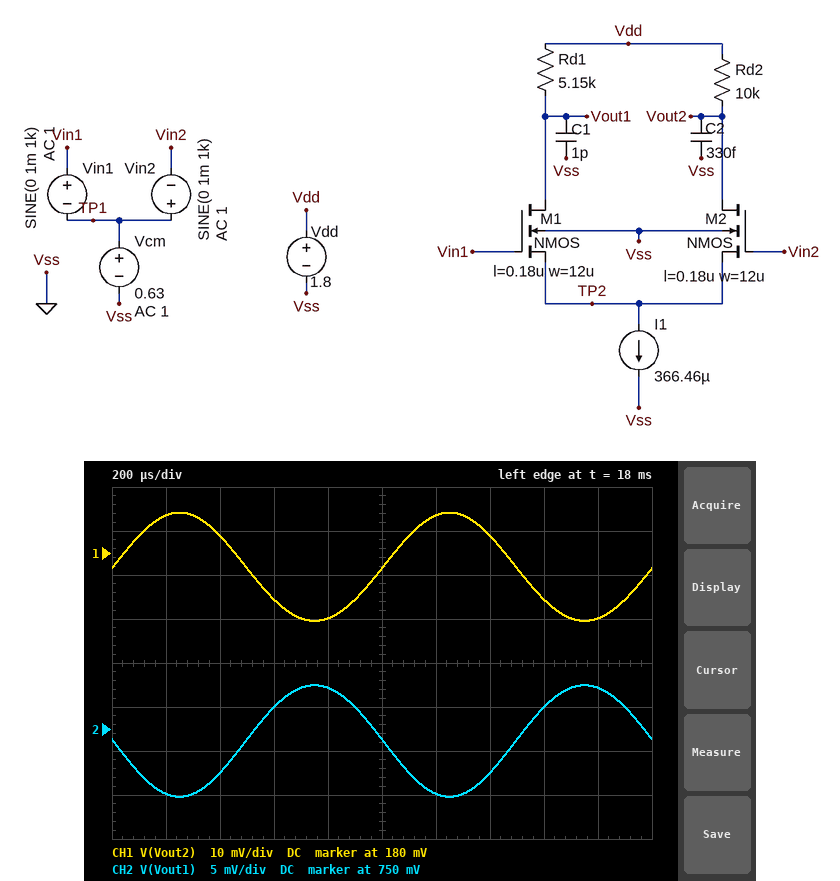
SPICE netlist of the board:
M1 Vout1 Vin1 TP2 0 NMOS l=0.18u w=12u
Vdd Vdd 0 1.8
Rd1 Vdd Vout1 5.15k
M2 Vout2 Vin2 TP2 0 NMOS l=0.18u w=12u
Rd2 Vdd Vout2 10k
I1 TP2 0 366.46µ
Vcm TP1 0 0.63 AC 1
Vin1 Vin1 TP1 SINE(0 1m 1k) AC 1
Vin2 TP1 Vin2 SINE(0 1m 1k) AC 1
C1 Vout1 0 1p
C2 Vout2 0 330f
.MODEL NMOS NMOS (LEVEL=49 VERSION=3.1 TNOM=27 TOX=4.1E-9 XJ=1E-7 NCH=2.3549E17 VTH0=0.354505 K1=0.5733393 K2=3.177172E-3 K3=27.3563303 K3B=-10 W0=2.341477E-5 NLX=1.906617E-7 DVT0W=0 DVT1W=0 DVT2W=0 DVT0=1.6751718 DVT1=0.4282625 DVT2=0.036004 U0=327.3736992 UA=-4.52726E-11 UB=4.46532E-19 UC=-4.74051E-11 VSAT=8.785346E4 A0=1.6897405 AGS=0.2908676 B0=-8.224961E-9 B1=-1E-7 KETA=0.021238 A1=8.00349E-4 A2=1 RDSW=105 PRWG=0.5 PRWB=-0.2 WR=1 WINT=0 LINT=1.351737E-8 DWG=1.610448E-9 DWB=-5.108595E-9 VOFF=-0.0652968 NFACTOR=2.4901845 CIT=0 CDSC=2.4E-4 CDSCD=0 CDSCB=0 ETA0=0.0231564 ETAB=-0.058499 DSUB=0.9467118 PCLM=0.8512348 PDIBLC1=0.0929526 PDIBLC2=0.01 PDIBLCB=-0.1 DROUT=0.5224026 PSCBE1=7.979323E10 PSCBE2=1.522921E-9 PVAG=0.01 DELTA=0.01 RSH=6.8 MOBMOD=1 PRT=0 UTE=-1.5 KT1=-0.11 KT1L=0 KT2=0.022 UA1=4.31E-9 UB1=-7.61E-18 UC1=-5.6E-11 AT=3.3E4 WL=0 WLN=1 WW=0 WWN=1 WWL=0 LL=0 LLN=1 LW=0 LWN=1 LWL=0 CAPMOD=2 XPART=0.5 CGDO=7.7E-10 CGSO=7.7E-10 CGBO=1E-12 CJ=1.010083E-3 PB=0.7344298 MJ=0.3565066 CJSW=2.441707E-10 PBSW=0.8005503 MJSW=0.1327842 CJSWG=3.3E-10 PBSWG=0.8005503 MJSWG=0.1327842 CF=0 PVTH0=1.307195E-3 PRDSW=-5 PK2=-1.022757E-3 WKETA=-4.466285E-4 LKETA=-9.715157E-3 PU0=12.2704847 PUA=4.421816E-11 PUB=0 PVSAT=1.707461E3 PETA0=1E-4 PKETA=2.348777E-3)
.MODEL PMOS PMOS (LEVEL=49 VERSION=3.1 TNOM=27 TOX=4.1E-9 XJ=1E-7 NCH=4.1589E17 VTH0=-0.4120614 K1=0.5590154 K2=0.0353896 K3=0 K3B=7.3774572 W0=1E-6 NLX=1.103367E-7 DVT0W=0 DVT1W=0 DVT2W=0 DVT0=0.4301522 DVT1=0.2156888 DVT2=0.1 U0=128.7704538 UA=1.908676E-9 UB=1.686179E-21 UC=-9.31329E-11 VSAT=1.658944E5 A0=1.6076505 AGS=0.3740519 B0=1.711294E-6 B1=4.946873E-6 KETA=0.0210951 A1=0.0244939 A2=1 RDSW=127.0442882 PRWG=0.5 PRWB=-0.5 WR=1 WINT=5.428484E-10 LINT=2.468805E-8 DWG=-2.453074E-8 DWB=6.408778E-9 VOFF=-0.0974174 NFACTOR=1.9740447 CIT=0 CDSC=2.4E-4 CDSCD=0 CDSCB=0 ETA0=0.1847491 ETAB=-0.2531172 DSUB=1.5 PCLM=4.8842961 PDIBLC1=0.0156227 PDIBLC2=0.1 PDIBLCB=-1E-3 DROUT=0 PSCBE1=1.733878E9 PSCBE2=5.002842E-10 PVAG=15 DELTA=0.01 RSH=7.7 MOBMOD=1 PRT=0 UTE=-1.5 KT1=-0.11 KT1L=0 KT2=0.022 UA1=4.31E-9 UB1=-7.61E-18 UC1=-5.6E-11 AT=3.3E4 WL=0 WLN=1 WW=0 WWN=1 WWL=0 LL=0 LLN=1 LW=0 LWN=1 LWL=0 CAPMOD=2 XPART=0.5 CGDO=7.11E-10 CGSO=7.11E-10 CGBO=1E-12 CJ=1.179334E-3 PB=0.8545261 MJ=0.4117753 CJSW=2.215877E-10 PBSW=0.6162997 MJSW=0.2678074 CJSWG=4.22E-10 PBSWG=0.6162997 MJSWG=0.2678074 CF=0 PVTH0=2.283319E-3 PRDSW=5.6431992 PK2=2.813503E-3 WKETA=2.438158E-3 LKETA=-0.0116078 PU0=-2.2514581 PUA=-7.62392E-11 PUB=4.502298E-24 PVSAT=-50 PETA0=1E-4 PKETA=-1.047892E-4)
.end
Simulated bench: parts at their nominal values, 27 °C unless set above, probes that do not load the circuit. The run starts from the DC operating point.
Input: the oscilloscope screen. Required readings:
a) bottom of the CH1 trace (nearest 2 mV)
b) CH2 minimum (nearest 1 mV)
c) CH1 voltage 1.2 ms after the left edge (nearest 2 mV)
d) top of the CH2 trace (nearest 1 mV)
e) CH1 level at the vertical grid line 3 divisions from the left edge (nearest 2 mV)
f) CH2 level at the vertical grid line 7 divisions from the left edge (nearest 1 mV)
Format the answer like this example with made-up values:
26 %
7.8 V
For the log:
164 mV
742 mV
188 mV
755 mV
170 mV
745 mV
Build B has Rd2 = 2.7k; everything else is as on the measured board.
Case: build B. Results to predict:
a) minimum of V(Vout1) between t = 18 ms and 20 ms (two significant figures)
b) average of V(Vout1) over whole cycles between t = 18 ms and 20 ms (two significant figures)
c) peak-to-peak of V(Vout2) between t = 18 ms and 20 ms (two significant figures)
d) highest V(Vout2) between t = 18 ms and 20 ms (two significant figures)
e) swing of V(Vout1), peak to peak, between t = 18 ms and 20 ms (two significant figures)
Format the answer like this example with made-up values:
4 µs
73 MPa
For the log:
900 mV
910 mV
11 mV
1.3 V
21 mV
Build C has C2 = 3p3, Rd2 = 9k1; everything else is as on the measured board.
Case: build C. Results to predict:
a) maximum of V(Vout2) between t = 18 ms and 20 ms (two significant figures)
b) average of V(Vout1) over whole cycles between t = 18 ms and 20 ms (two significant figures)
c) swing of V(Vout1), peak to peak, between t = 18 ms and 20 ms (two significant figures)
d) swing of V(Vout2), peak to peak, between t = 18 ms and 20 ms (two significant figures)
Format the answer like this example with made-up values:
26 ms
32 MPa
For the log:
290 mV
770 mV
16 mV
28 mV
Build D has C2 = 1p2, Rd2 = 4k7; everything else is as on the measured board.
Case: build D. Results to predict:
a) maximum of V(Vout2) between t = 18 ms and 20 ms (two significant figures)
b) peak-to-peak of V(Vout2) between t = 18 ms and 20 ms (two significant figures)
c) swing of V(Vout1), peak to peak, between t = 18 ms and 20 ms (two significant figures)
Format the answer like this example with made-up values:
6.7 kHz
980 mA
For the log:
940 mV
18 mV
20 mV
